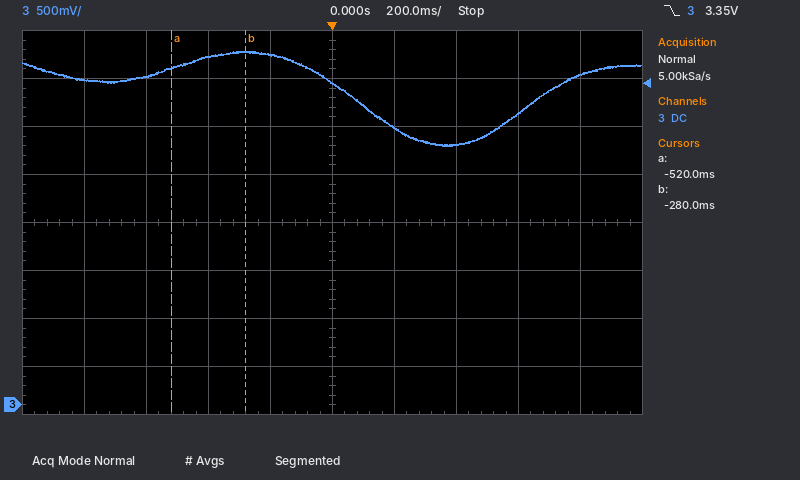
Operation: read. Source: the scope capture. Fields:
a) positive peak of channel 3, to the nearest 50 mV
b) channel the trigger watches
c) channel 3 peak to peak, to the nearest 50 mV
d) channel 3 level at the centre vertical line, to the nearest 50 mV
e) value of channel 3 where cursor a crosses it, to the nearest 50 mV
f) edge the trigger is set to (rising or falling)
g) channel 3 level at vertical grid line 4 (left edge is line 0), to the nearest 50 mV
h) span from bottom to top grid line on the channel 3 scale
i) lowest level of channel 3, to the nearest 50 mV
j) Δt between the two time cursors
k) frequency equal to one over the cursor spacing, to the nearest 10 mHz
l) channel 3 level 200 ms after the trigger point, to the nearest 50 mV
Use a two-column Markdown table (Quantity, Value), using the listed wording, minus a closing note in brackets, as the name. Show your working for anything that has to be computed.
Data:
| Quantity | Value |
|---|---|
| positive peak of channel 3, to the nearest 50 mV | 3.70 V |
| channel the trigger watches | channel 3 |
| channel 3 peak to peak, to the nearest 50 mV | 3.70 V − (2.70 V) = 1.00 V |
| channel 3 level at the centre vertical line, to the nearest 50 mV | 3.35 V |
| value of channel 3 where cursor a crosses it, to the nearest 50 mV | 3.50 V |
| edge the trigger is set to | falling |
| channel 3 level at vertical grid line 4 (left edge is line 0), to the nearest 50 mV | 3.65 V |
| span from bottom to top grid line on the channel 3 scale | 4 V |
| lowest level of channel 3, to the nearest 50 mV | 2.70 V |
| Δt between the two time cursors | -280 ms − (-520 ms) = 240 ms |
| frequency equal to one over the cursor spacing, to the nearest 10 mHz | 1 / 240 ms ≈ 4.17 Hz |
| channel 3 level 200 ms after the trigger point, to the nearest 50 mV | 2.90 V |
